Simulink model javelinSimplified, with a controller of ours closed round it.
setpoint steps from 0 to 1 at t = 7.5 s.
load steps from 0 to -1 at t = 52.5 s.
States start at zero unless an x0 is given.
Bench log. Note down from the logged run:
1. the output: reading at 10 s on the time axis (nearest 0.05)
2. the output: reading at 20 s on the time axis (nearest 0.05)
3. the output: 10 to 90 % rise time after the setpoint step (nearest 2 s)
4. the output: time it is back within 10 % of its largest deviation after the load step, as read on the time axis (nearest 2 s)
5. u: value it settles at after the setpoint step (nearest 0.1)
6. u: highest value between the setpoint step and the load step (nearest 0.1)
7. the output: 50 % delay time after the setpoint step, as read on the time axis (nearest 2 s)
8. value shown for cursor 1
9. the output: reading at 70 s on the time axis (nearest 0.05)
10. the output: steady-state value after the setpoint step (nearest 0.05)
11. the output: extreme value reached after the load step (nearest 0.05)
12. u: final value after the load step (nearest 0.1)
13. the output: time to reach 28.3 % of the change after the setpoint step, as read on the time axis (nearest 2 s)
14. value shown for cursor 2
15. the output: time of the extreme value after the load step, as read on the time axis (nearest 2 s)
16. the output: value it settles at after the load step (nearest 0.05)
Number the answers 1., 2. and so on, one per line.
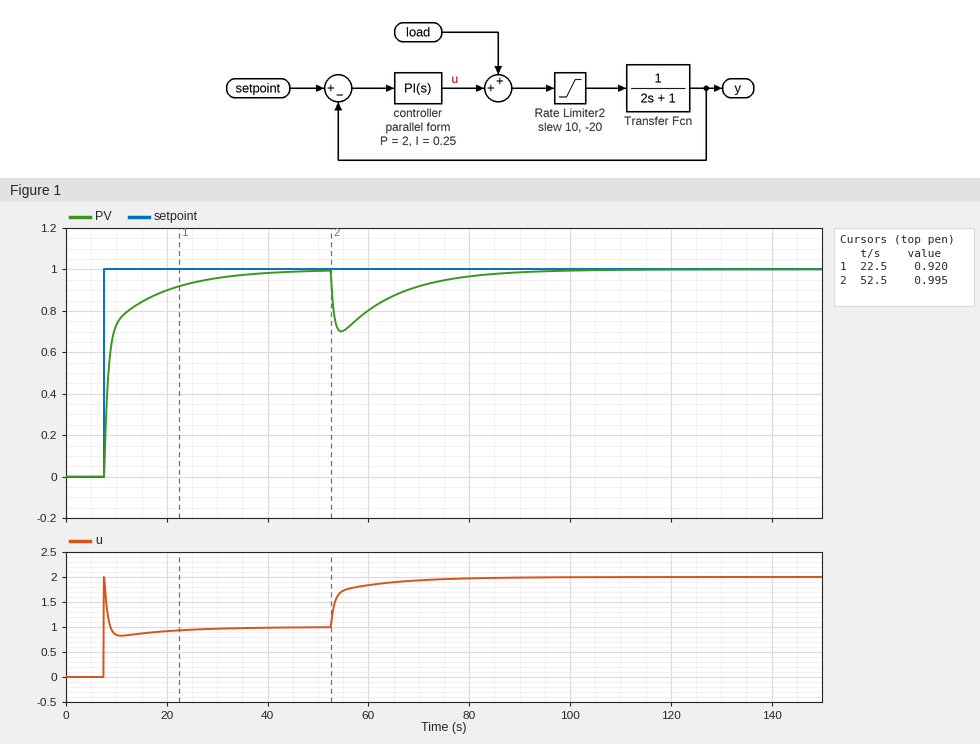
1. 0.75
2. 0.90
3. 12 s
4. 82 s
5. 1.0
6. 2.0
7. 8 s
8. 0.920
9. 0.90
10. 1.00
11. 0.70
12. 2.0
13. 8 s
14. 0.995
15. 54 s
16. 1.00
